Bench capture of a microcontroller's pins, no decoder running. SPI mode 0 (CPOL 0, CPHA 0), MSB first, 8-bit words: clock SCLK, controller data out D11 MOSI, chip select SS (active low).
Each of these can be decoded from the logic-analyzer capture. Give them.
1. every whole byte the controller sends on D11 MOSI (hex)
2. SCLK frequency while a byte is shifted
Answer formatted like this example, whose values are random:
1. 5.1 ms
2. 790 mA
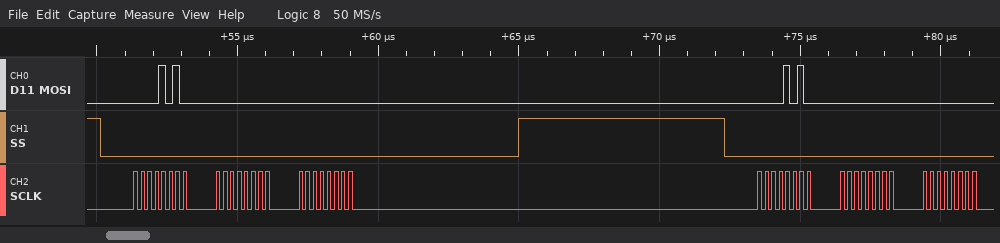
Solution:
1. 0x0A 0x00 0x00 0x0A 0x00 0x00
2. 4 MHz
